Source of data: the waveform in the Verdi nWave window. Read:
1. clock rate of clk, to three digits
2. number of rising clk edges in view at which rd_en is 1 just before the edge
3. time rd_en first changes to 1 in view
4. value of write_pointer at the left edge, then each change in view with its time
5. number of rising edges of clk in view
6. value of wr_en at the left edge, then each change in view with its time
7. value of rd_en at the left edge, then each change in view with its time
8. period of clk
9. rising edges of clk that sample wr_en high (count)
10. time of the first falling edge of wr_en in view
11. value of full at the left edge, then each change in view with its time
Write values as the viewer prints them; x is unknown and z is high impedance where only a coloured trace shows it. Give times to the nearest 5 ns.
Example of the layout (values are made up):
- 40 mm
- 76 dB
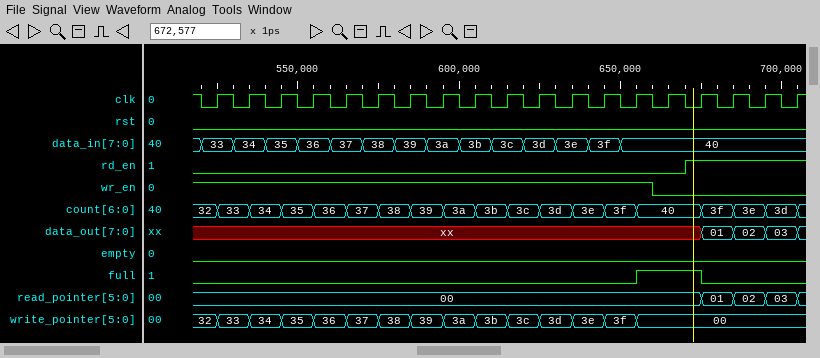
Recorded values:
- 100 MHz
- 4
- 670 ns
- 32, 33 at 525 ns, 34 at 535 ns, 35 at 545 ns, 36 at 555 ns, 37 at 565 ns, 38 at 575 ns, 39 at 585 ns, 3a at 595 ns, 3b at 605 ns, 3c at 615 ns, 3d at 625 ns, 3e at 635 ns, 3f at 645 ns, 00 at 655 ns
- 19
- 1, 0 at 660 ns
- 0, 1 at 670 ns
- 10 ns
- 14
- 660 ns
- 0, 1 at 655 ns, 0 at 675 ns
